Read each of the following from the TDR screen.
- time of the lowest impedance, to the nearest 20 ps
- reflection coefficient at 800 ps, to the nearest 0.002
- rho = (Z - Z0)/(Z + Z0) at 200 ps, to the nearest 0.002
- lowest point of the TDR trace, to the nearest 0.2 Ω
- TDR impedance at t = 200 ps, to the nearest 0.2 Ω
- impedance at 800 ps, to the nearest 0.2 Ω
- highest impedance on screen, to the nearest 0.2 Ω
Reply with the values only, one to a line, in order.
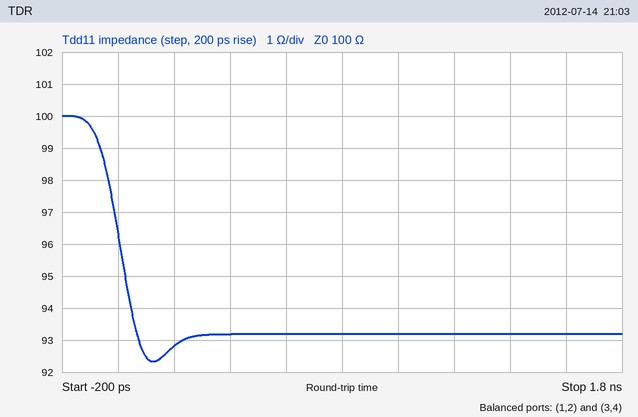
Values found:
120 ps
-0.036
-0.038
92.4 Ω
92.8 Ω
93.2 Ω
100.0 Ω
